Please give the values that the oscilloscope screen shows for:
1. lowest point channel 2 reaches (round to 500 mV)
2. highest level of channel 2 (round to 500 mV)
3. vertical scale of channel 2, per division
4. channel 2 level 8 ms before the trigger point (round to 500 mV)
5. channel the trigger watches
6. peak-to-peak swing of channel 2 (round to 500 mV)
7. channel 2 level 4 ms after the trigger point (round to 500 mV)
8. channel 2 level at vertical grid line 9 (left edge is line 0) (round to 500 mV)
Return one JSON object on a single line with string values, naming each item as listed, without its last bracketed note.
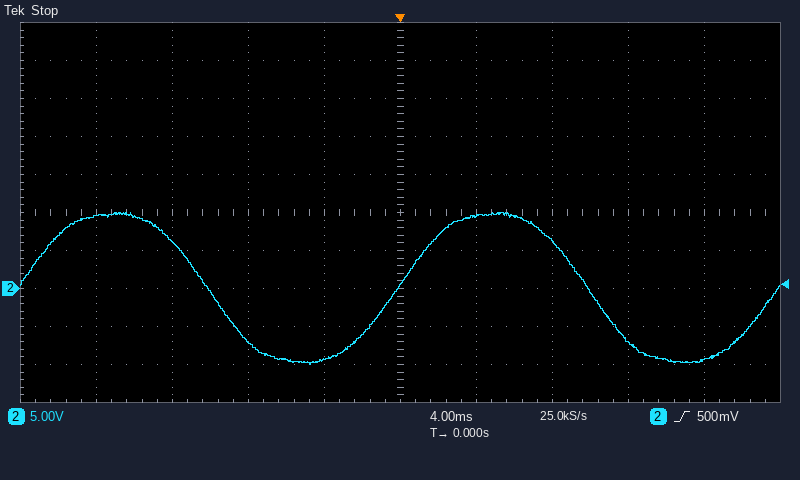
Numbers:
{"lowest point channel 2 reaches": "-10.0 V", "highest level of channel 2": "10.0 V", "vertical scale of channel 2, per division": "5 V", "channel 2 level 8 ms before the trigger point": "-7.0 V", "channel the trigger watches": "channel 2", "peak-to-peak swing of channel 2": "20.0 V", "channel 2 level 4 ms after the trigger point": "9.5 V", "channel 2 level at vertical grid line 9 (left edge is line 0)": "-9.5 V"}
